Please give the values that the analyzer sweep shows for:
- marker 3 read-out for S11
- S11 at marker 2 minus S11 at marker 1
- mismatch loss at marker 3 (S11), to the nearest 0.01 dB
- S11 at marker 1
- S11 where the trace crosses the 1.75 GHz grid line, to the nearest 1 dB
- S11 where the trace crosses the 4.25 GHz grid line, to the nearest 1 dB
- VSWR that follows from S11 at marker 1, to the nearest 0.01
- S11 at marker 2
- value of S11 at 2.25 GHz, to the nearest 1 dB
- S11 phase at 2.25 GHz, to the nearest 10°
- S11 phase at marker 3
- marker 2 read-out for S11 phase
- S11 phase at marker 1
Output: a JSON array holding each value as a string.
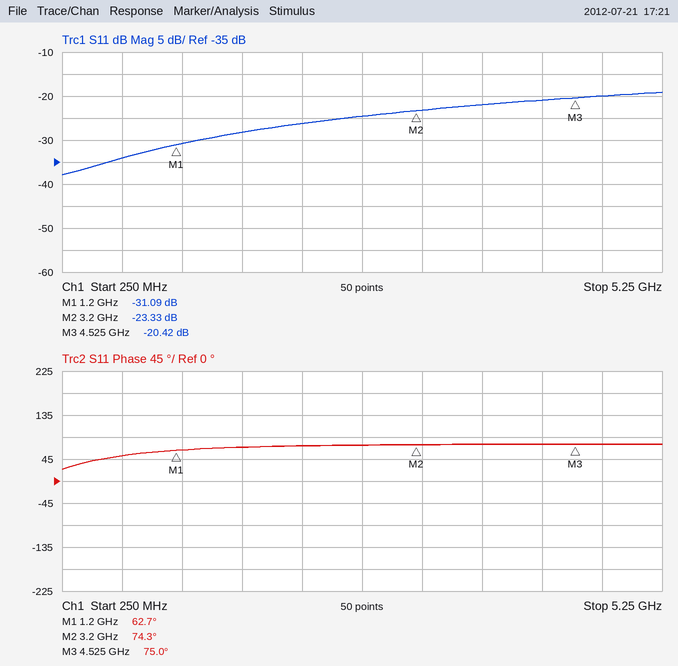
["-20.42 dB", "7.76 dB", "0.04 dB", "-31.09 dB", "-28 dB", "-21 dB", "1.06", "-23.33 dB", "-26 dB", "70°", "75.0°", "74.3°", "62.7°"]
